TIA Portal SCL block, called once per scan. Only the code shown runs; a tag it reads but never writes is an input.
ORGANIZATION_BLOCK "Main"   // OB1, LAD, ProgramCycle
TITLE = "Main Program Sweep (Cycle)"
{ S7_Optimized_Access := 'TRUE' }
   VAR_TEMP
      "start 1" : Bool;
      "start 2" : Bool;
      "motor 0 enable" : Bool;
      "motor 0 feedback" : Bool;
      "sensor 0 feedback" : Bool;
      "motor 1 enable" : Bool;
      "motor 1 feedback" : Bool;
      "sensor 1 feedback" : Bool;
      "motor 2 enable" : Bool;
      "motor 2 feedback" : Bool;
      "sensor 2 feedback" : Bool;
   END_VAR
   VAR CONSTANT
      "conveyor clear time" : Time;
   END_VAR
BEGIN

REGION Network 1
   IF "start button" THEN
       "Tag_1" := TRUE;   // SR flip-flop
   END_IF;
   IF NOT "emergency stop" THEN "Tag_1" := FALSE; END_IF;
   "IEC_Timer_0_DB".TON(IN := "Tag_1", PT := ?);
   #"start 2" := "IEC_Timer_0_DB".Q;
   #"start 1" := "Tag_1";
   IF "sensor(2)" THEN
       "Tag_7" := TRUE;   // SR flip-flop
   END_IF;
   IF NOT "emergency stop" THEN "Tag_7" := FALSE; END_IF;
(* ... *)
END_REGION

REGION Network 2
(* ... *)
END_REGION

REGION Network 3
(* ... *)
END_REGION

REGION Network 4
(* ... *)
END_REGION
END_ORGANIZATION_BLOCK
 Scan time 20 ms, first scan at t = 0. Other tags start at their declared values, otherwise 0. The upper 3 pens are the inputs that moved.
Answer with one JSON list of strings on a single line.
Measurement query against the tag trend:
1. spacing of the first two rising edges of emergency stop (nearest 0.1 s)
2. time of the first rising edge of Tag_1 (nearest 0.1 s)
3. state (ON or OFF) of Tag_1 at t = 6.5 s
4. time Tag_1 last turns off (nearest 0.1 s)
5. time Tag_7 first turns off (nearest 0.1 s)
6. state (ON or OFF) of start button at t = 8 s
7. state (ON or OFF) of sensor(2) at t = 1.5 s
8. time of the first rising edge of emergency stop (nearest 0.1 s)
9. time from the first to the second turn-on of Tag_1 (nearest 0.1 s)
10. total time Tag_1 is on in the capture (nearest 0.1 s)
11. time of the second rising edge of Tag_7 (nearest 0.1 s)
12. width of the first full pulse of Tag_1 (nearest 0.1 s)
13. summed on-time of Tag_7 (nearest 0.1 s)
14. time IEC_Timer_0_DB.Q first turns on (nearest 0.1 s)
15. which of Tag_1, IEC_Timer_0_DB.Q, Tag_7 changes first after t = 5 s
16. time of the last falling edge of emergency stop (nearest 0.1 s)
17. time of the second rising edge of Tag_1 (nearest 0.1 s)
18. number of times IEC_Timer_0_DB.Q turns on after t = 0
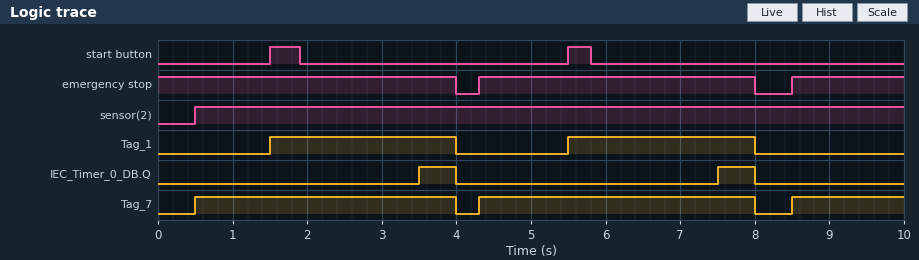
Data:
["4.2 s", "1.5 s", "ON", "8.0 s", "4.0 s", "OFF", "ON", "4.3 s", "4.0 s", "5.0 s", "4.3 s", "2.5 s", "8.7 s", "3.5 s", "Tag_1", "8.0 s", "5.5 s", "2"]
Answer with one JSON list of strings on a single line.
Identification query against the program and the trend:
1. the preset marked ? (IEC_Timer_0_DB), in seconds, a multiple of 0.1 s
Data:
["2.0 s"]
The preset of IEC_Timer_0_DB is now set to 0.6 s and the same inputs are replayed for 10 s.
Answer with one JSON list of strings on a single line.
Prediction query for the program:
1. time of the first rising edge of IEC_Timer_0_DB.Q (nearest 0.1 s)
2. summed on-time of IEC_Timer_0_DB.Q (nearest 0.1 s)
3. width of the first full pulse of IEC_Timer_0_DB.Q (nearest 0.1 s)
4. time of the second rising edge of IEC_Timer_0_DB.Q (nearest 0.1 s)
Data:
["2.1 s", "3.8 s", "1.9 s", "6.1 s"]
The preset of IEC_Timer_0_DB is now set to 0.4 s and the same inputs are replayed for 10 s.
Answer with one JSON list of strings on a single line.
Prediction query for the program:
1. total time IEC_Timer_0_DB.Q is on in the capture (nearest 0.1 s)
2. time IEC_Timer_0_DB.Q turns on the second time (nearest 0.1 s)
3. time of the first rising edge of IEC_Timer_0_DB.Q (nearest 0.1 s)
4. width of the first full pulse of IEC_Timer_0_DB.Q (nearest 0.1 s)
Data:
["4.2 s", "5.9 s", "1.9 s", "2.1 s"]
